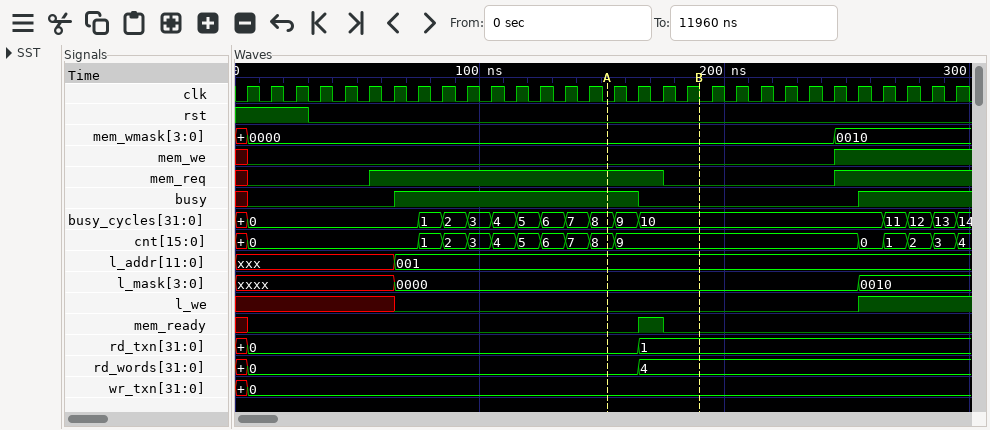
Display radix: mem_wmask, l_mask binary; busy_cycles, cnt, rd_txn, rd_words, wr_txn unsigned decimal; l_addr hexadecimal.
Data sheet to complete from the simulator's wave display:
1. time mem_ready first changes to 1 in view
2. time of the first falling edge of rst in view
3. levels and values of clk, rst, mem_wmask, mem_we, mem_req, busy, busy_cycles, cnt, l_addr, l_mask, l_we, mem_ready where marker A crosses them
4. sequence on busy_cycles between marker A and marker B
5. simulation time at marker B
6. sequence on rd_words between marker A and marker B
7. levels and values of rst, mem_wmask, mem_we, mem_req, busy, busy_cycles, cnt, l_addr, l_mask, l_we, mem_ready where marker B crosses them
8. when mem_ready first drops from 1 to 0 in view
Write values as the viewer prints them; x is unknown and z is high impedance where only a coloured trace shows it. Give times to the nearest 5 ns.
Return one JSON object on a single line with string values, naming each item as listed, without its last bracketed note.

{"time mem_ready first changes to 1 in view": "165 ns", "time of the first falling edge of rst in view": "30 ns", "levels and values of clk, rst, mem_wmask, mem_we, mem_req, busy, busy_cycles, cnt, l_addr, l_mask, l_we, mem_ready where marker A crosses them": "clk=0, rst=0, mem_wmask=0000, mem_we=0, mem_req=1, busy=1, busy_cycles=8, cnt=8, l_addr=001, l_mask=0000, l_we=0, mem_ready=0", "sequence on busy_cycles between marker A and marker B": "8, 9, 10", "simulation time at marker B": "190 ns", "sequence on rd_words between marker A and marker B": "0, 4", "levels and values of rst, mem_wmask, mem_we, mem_req, busy, busy_cycles, cnt, l_addr, l_mask, l_we, mem_ready where marker B crosses them": "rst=0, mem_wmask=0000, mem_we=0, mem_req=0, busy=0, busy_cycles=10, cnt=9, l_addr=001, l_mask=0000, l_we=0, mem_ready=0", "when mem_ready first drops from 1 to 0 in view": "175 ns"}
